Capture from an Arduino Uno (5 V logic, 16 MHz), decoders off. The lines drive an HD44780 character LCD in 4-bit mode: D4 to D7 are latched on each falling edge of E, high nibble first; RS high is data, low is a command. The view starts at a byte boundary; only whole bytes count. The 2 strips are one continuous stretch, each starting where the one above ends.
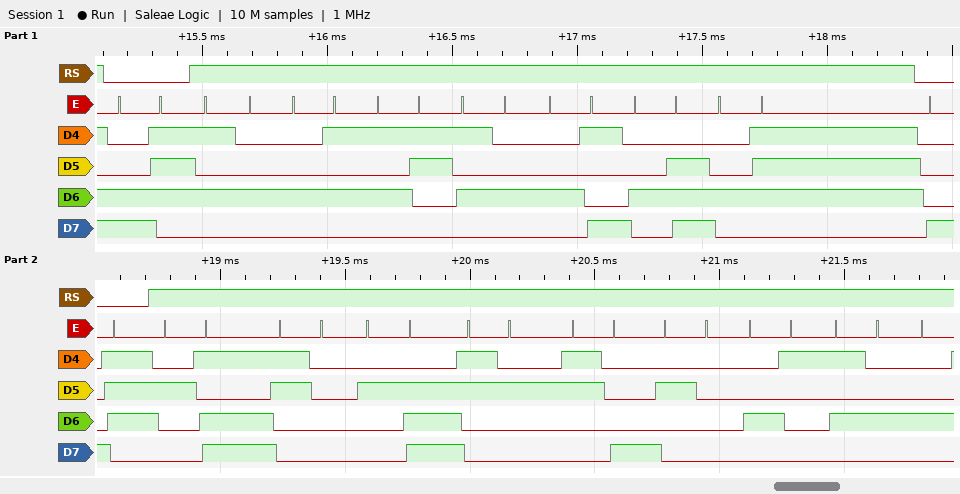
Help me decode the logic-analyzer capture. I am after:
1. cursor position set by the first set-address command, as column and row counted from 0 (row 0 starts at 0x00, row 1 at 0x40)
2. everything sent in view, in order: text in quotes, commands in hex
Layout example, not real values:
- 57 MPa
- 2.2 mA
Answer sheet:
- column 7, row 1
- 0xC7 "TESTING" 0x87 "-0.28 AT"
